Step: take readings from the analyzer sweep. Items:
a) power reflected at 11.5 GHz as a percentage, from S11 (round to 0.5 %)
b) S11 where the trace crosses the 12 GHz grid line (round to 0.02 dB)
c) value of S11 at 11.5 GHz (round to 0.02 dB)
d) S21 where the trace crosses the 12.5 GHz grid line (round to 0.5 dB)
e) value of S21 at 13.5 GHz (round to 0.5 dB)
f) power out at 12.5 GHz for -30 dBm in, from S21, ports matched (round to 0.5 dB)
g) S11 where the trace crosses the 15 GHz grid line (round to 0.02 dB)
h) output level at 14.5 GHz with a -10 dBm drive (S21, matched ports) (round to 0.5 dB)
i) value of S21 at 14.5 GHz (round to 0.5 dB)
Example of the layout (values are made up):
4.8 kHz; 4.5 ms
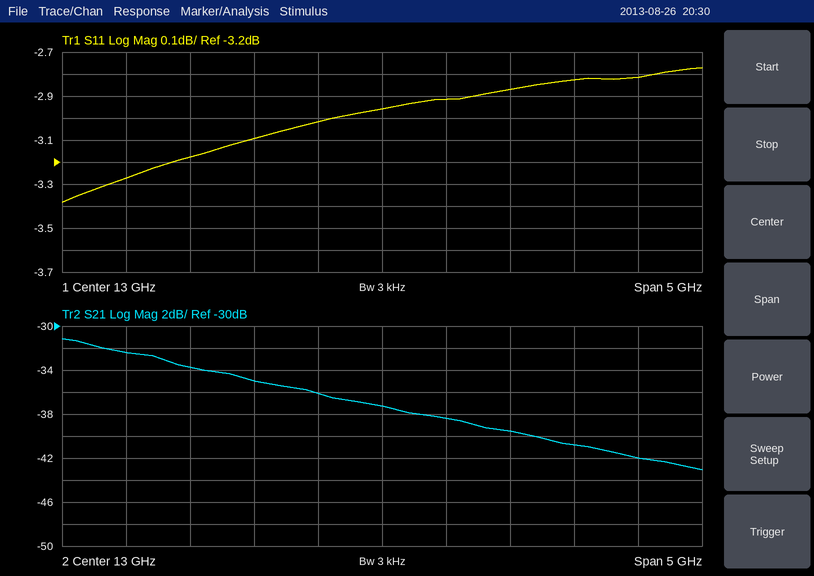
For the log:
48.0 %; -3.10 dB; -3.18 dB; -36.0 dB; -38.5 dB; -66.0 dBm; -2.82 dB; -51.0 dBm; -41.0 dB
